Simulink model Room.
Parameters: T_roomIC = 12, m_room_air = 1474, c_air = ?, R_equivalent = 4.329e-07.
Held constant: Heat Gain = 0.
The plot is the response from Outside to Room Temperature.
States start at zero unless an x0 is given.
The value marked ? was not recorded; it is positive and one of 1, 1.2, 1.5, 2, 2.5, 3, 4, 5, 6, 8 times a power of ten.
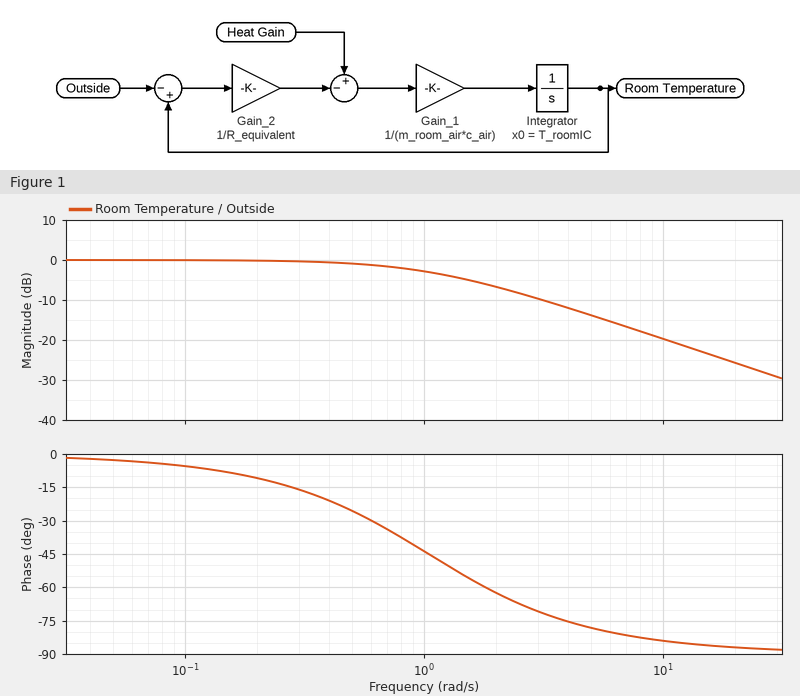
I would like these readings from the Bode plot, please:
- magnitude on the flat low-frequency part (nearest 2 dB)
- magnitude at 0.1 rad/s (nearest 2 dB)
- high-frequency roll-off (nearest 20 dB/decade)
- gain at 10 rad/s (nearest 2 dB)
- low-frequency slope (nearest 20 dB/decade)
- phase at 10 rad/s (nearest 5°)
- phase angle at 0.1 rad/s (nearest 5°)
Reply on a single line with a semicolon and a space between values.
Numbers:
0 dB; 0 dB; -20 dB/decade; -20 dB; 0 dB/decade; -85°; -5°
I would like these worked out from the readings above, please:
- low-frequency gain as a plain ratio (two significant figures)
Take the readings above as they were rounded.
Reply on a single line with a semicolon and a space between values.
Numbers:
1.0
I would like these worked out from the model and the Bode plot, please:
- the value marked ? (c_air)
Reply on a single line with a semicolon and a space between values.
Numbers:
1500
